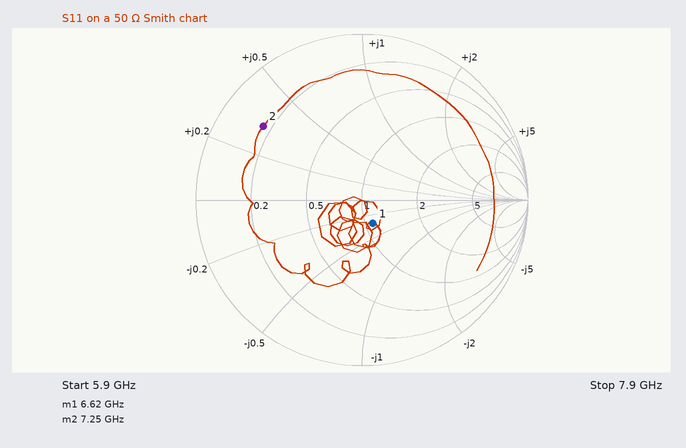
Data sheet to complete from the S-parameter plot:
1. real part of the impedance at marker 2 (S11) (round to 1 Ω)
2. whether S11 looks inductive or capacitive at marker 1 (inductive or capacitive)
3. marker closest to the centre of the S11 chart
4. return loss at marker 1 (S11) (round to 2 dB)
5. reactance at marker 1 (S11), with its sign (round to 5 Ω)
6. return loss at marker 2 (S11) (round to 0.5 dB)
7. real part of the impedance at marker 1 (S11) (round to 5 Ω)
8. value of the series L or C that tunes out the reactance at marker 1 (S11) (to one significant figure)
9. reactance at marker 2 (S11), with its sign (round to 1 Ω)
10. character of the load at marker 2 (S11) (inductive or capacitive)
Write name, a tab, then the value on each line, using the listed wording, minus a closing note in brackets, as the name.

real part of the impedance at marker 2 (S11)	8 Ω
whether S11 looks inductive or capacitive at marker 1	capacitive
marker closest to the centre of the S11 chart	marker 1
return loss at marker 1 (S11)	16 dB
reactance at marker 1 (S11), with its sign	-15 Ω
return loss at marker 2 (S11)	2.5 dB
real part of the impedance at marker 1 (S11)	55 Ω
value of the series L or C that tunes out the reactance at marker 1 (S11)	400 pH
reactance at marker 2 (S11), with its sign	+16 Ω
character of the load at marker 2 (S11)	inductive
